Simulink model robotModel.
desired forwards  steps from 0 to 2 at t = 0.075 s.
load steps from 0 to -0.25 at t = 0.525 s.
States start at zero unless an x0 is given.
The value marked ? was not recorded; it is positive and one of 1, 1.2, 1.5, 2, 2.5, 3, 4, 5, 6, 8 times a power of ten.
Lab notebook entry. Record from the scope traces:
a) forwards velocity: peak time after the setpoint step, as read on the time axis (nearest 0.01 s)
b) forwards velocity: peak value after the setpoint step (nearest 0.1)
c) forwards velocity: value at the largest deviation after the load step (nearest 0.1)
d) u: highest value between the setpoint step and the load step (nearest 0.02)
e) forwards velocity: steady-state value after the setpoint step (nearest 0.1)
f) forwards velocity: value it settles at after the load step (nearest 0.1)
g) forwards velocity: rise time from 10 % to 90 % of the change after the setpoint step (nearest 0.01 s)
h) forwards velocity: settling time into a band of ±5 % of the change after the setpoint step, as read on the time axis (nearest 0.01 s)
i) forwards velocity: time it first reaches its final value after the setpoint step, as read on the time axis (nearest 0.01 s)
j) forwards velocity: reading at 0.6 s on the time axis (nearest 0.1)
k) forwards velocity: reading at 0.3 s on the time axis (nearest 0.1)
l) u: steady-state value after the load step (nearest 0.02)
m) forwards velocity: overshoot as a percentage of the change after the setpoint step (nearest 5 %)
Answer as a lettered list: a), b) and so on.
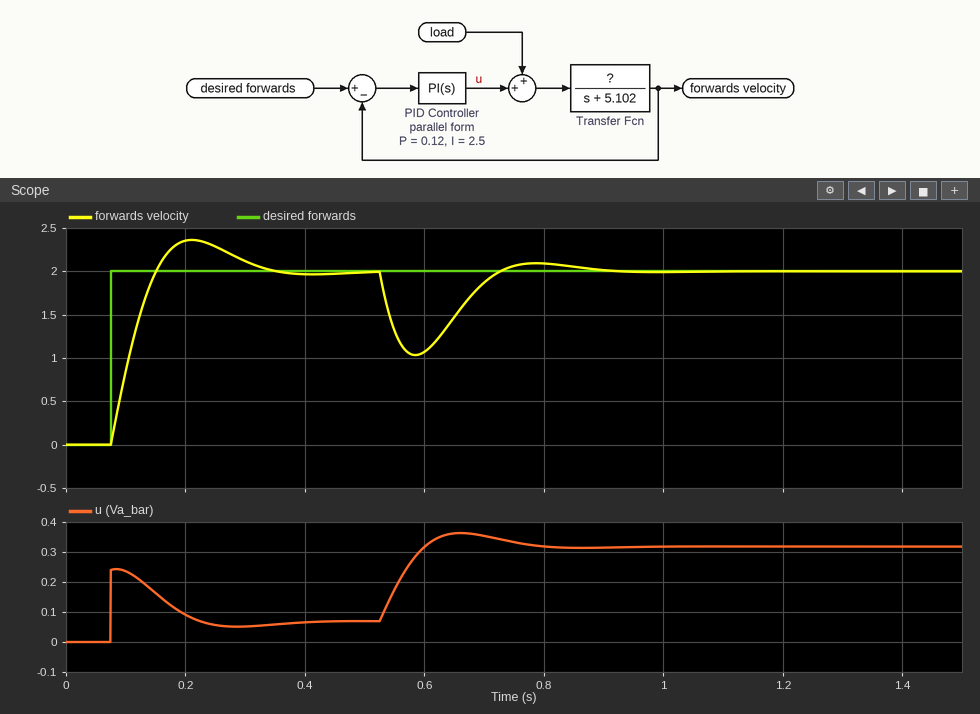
a) 0.21 s
b) 2.4
c) 1.0
d) 0.24
e) 2.0
f) 2.0
g) 0.06 s
h) 0.31 s
i) 0.15 s
j) 1.1
k) 2.1
l) 0.32
m) 20 %
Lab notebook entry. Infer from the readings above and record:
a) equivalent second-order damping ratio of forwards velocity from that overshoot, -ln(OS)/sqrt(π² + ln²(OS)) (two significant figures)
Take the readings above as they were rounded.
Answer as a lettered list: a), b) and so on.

a) 0.46
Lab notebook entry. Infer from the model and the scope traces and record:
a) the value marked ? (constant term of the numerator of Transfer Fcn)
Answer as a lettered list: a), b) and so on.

a) 150
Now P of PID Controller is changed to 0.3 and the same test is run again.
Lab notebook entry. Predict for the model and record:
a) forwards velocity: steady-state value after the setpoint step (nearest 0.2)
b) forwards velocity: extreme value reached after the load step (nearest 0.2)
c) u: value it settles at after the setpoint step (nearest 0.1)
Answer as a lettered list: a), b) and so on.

a) 2.0
b) 1.4
c) 0.1
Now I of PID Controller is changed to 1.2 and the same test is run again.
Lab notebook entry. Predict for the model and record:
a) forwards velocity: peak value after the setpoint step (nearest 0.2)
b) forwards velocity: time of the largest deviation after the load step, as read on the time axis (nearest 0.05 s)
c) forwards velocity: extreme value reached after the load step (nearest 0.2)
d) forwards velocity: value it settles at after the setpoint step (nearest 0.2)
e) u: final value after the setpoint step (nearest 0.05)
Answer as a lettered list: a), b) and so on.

a) 2.2
b) 0.60 s
c) 0.8
d) 2.0
e) 0.05
